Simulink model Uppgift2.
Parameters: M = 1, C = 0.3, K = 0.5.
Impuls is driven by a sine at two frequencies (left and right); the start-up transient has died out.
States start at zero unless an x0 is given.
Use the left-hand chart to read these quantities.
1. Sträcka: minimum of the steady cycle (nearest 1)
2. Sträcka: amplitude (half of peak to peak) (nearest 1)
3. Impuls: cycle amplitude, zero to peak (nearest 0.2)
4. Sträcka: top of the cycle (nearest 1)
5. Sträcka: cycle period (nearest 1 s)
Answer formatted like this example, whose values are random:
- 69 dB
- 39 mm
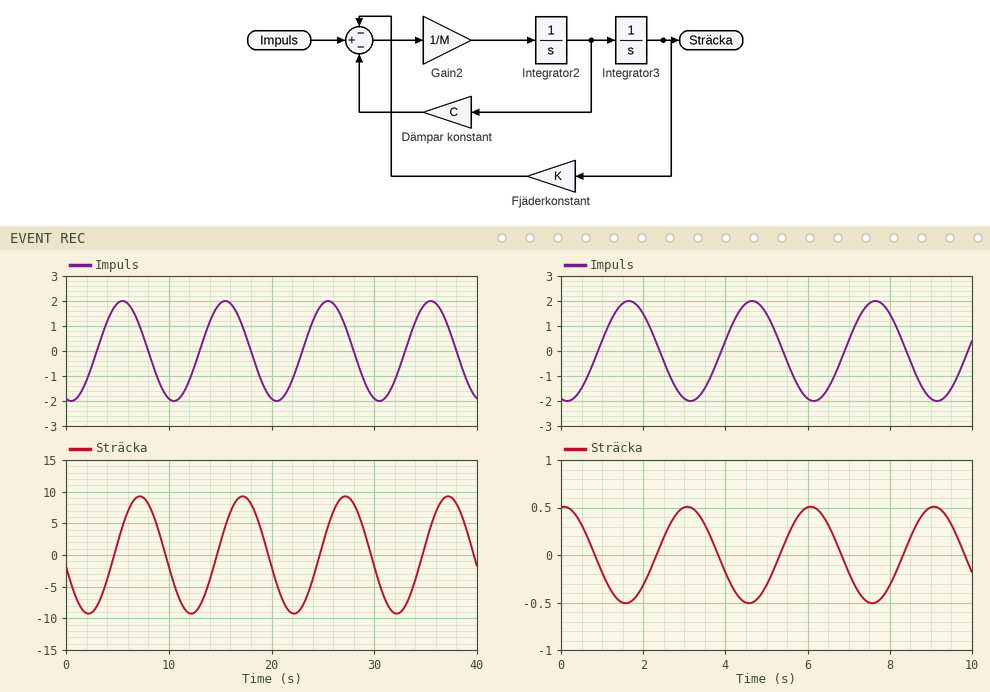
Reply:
- -9
- 9
- 2.0
- 9
- 10 s
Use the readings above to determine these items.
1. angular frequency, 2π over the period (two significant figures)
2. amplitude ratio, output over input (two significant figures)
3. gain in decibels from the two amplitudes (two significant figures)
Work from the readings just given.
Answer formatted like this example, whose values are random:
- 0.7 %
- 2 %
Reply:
- 0.63 rad/s
- 4.5
- 13 dB
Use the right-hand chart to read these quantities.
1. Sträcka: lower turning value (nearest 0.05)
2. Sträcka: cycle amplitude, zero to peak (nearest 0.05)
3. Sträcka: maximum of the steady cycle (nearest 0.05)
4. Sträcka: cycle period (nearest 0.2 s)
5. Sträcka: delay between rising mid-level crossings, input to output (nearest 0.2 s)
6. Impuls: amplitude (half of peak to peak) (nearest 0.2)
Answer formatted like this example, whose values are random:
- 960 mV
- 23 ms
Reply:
- -0.50
- 0.50
- 0.50
- 3.0 s
- 1.4 s
- 2.0
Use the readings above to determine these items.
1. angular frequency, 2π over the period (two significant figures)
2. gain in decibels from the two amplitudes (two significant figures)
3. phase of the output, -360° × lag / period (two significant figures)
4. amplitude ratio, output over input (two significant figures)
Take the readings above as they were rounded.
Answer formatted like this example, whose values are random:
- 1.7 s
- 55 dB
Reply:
- 2.1 rad/s
- -12 dB
- -170°
- 0.25
